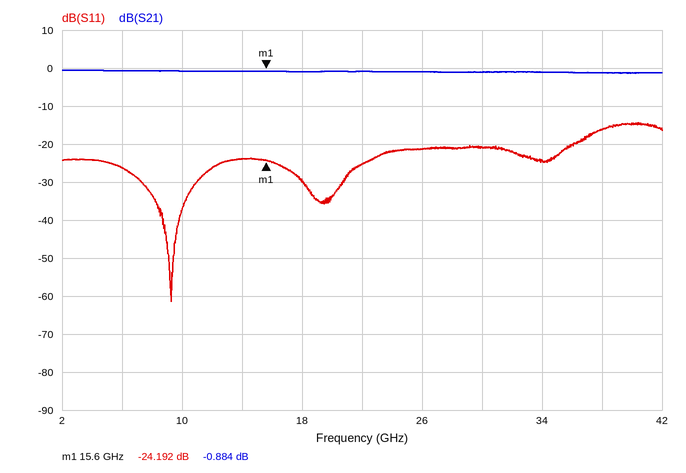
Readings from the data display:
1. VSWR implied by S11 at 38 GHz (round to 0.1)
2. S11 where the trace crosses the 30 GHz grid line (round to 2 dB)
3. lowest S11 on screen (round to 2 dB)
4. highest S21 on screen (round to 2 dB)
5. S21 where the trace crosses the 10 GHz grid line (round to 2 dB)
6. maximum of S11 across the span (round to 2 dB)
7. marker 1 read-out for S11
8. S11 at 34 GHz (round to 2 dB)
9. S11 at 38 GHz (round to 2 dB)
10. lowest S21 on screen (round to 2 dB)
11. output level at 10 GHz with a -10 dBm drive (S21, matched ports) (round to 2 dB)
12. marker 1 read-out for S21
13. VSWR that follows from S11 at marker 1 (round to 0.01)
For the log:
1.4
-20 dB
-62 dB
0 dB
0 dB
-14 dB
-24.192 dB
-24 dB
-16 dB
-2 dB
-10 dBm
-0.884 dB
1.13
